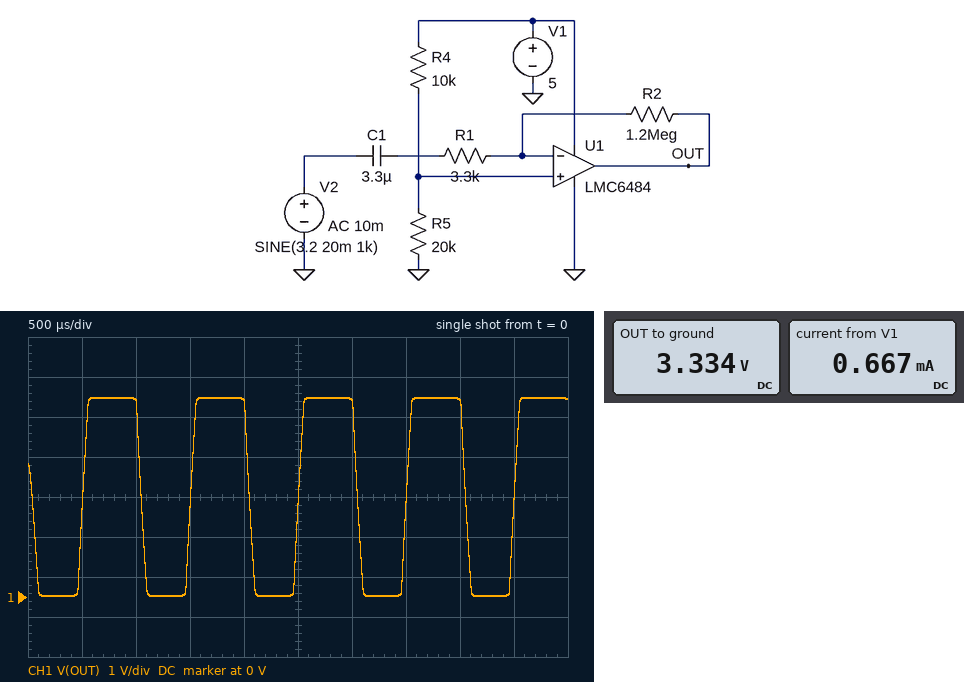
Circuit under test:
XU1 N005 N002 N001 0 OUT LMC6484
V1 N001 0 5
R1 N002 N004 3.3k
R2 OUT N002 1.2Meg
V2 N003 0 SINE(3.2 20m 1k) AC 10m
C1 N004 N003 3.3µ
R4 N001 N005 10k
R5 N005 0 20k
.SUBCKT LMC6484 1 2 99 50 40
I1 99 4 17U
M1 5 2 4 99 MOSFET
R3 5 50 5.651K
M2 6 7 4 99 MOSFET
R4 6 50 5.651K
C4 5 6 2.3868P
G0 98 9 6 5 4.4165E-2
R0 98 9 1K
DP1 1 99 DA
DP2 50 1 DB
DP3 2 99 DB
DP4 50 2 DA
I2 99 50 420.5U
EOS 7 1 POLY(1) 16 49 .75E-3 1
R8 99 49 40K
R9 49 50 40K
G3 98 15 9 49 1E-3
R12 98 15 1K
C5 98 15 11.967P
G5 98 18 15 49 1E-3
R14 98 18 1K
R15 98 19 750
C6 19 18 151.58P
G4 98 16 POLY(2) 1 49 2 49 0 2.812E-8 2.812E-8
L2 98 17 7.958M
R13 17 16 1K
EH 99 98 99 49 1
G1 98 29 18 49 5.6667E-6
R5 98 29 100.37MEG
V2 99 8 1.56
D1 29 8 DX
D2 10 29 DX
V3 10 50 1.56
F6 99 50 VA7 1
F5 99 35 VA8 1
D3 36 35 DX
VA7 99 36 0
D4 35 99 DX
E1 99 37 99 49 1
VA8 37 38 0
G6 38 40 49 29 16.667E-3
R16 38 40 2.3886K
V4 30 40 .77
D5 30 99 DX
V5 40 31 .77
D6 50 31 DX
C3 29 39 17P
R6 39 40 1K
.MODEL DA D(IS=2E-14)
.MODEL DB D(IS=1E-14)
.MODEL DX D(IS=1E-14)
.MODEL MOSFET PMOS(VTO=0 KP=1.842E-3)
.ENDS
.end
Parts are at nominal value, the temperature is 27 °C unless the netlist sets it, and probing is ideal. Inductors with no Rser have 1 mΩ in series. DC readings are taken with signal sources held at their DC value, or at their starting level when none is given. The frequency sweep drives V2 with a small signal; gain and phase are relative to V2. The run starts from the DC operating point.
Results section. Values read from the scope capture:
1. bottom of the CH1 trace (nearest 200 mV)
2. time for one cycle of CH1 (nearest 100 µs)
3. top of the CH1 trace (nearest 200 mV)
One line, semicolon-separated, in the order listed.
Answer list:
0 V; 1.0 ms; 5.0 V
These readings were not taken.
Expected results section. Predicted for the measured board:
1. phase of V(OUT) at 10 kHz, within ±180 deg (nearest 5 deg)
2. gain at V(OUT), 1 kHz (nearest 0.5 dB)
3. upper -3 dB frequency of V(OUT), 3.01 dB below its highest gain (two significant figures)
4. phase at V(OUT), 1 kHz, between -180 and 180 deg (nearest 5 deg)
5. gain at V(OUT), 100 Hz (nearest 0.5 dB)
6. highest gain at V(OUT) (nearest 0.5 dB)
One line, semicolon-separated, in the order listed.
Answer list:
120 deg; 51.0 dB; 6.3 kHz; 170 deg; 51.0 dB; 51.0 dB
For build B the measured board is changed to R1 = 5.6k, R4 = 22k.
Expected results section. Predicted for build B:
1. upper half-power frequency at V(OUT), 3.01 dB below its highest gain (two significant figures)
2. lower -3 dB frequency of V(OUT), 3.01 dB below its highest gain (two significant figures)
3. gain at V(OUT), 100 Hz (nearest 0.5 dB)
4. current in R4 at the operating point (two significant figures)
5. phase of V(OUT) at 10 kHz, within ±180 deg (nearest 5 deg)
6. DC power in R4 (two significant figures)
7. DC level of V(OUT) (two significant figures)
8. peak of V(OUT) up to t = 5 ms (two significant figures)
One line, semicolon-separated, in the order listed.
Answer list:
11 kHz; 8.6 Hz; 46.5 dB; 120 µA; 135 deg; 310 µW; 2.4 V; 5.0 V
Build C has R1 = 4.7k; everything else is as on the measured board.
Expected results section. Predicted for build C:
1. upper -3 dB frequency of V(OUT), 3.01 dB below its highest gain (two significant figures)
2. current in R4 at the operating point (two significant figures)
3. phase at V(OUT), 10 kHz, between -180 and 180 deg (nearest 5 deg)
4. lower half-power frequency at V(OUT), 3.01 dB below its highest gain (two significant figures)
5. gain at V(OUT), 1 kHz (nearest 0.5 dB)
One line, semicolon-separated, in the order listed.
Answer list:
9.0 kHz; 170 µA; 130 deg; 10 Hz; 48.0 dB
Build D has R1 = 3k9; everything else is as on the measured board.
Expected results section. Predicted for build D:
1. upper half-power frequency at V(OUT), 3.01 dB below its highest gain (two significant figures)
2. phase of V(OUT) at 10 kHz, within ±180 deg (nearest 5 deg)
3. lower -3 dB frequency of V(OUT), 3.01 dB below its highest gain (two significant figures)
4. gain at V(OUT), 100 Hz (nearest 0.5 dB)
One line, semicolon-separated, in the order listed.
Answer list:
7.5 kHz; 125 deg; 12 Hz; 49.5 dB
